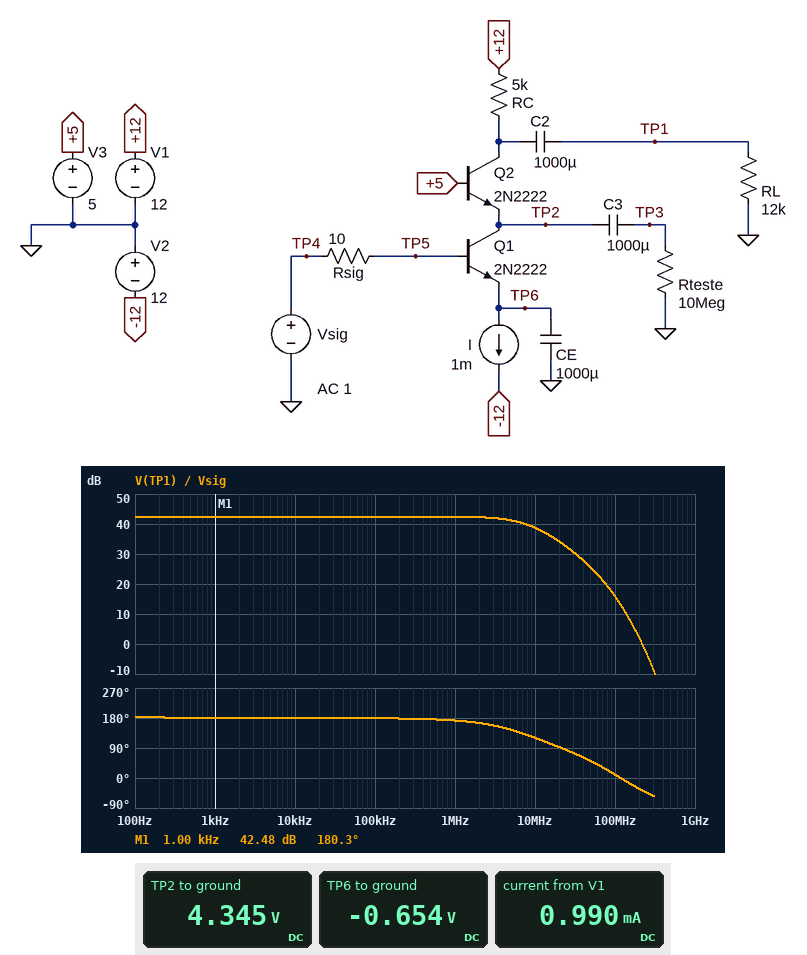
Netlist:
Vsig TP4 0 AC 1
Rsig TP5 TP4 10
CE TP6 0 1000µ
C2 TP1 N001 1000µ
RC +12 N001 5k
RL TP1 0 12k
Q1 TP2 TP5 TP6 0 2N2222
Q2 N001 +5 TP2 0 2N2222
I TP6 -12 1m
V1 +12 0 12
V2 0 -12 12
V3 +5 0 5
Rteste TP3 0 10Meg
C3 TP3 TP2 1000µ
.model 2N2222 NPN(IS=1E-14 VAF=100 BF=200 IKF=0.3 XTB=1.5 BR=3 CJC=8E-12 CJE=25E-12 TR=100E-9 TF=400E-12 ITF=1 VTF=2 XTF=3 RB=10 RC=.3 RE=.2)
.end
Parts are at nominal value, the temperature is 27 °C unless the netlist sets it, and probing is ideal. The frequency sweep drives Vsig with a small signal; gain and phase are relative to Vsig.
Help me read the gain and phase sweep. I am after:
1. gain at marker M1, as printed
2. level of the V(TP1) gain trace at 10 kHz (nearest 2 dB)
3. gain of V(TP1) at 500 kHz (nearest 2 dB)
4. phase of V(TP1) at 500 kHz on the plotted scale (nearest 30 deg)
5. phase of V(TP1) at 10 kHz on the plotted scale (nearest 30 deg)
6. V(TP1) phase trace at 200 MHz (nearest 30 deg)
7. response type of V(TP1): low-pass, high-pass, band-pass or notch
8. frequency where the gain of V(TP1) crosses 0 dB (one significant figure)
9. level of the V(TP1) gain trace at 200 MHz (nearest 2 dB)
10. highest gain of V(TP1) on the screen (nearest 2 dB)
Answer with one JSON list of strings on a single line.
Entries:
["42.48 dB", "42 dB", "42 dB", "180 deg", "180 deg", "-30 deg", "low-pass", "200 MHz", "2 dB", "42 dB"]
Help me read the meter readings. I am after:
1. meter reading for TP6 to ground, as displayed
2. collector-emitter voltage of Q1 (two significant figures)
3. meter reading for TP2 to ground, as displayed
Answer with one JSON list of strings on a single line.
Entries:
["-0.654 V", "5.0 V", "4.345 V"]
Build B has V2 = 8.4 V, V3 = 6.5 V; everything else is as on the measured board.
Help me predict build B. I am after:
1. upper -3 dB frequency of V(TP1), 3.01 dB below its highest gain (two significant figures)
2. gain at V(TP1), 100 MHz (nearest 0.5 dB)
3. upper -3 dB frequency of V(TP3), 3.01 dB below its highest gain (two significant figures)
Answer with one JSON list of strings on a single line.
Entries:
["6.7 MHz", "13.5 dB", "81 MHz"]
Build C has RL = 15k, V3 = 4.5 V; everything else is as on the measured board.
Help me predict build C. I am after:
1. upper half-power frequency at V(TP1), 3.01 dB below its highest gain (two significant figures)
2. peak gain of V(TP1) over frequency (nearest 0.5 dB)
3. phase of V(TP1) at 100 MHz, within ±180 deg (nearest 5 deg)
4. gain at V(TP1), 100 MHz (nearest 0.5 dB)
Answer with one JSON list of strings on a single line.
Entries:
["8.5 MHz", "43.0 dB", "10 deg", "16.5 dB"]
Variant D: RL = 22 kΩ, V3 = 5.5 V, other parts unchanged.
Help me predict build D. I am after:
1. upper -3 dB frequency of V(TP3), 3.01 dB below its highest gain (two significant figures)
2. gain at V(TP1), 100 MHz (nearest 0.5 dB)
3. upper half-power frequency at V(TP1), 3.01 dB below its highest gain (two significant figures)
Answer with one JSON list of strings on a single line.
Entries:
["81 MHz", "15.5 dB", "7.0 MHz"]
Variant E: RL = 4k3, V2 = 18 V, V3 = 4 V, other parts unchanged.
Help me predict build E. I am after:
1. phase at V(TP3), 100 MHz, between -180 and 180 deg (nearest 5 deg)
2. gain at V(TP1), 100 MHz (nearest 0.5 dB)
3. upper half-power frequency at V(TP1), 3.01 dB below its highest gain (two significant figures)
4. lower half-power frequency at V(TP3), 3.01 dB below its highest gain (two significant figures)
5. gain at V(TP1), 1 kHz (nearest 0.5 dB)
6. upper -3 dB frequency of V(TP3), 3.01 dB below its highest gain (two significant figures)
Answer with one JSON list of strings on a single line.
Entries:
["110 deg", "16.5 dB", "14 MHz", "10 Hz", "39.0 dB", "86 MHz"]
